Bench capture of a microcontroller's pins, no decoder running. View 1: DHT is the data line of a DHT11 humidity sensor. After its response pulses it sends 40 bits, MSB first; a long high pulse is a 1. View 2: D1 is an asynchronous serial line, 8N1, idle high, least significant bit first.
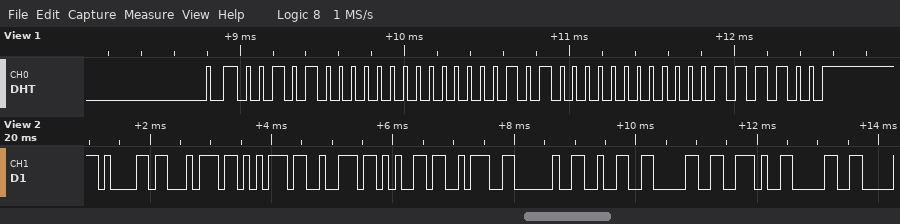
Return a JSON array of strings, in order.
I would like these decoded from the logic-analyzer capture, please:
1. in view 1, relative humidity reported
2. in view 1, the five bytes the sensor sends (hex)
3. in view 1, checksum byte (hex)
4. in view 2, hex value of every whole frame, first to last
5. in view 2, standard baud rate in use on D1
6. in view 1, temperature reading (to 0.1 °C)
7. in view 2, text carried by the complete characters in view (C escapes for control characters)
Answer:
["40 %", "28 00 14 00 3C", "0x3C", "61 74 75 72 65 3A 20 32 30 2E 30", "9600 baud", "20.0 °C", "\"ature: 20.0\""]
